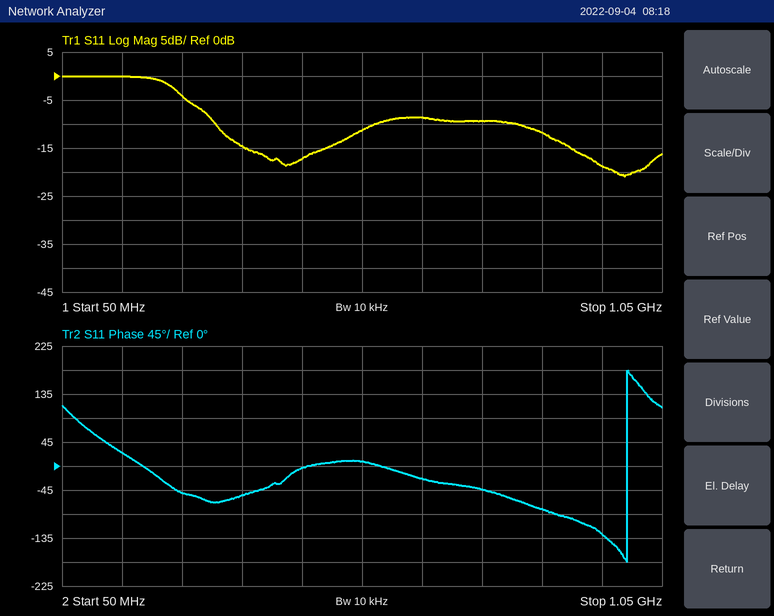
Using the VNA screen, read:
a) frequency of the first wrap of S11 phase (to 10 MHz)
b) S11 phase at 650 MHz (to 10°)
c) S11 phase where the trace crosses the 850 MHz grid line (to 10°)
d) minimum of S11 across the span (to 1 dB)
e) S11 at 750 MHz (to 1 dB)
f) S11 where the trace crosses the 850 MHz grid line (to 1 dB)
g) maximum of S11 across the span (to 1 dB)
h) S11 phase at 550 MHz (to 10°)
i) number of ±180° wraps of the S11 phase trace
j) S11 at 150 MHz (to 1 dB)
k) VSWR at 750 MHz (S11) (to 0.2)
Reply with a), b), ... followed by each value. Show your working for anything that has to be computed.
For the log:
a) 990 MHz
b) -20°
c) -80°
d) -21 dB
e) -9 dB
f) -12 dB
g) 0 dB
h) 10°
i) 1
j) 0 dB
k) |Γ| = 10^(-9/20) = 0.3548; VSWR = (1 + 0.3548)/(1 − 0.3548) ≈ 2.10, so 2.0 to the nearest 0.2
